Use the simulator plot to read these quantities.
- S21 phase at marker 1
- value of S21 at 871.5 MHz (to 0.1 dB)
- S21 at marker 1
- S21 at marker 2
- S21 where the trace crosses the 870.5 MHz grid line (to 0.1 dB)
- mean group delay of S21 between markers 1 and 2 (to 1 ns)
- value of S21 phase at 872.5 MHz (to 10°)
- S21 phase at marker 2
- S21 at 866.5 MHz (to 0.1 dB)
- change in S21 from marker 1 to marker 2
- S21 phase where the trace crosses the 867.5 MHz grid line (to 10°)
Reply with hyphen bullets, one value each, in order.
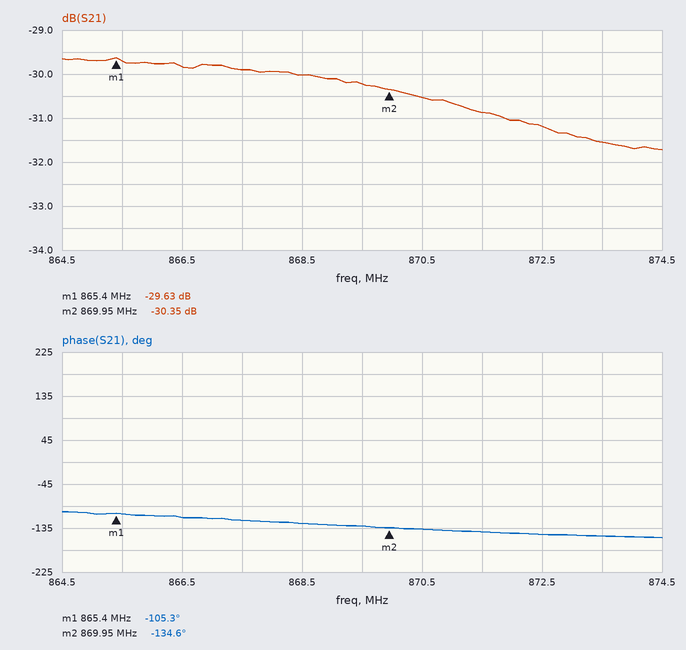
- -105.3°
- -30.9 dB
- -29.63 dB
- -30.35 dB
- -30.5 dB
- 18 ns
- -150°
- -134.6°
- -29.8 dB
- -0.72 dB
- -120°
